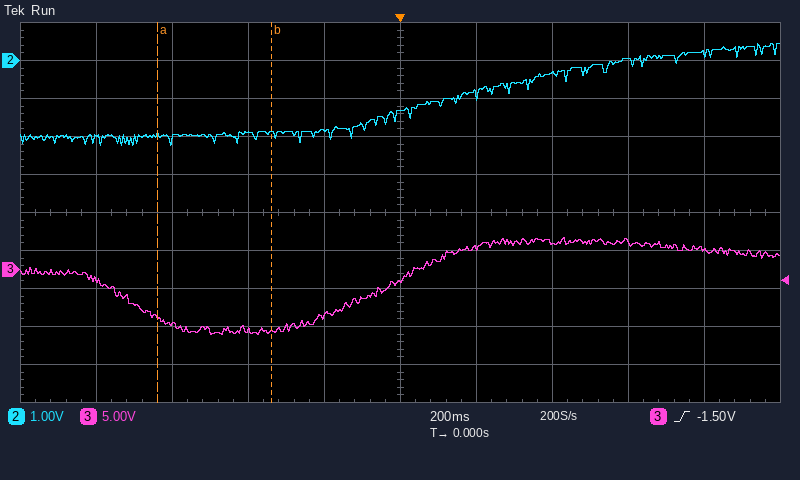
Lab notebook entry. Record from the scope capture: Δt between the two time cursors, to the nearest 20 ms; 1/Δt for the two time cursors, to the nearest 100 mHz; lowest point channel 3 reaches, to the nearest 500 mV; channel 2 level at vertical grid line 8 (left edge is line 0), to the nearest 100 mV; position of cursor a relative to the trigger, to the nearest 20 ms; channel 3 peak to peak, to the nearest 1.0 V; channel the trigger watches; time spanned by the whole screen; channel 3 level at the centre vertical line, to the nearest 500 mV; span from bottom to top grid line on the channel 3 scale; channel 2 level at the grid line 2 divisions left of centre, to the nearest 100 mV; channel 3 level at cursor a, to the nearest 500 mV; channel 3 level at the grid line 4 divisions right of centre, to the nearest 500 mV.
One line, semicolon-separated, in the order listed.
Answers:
300 ms; 3.3 Hz; -8.5 V; 0.0 V; -640 ms; 13.0 V; channel 3; 2 s; -1.5 V; 50 V; -1.9 V; -6.5 V; 2.5 V
